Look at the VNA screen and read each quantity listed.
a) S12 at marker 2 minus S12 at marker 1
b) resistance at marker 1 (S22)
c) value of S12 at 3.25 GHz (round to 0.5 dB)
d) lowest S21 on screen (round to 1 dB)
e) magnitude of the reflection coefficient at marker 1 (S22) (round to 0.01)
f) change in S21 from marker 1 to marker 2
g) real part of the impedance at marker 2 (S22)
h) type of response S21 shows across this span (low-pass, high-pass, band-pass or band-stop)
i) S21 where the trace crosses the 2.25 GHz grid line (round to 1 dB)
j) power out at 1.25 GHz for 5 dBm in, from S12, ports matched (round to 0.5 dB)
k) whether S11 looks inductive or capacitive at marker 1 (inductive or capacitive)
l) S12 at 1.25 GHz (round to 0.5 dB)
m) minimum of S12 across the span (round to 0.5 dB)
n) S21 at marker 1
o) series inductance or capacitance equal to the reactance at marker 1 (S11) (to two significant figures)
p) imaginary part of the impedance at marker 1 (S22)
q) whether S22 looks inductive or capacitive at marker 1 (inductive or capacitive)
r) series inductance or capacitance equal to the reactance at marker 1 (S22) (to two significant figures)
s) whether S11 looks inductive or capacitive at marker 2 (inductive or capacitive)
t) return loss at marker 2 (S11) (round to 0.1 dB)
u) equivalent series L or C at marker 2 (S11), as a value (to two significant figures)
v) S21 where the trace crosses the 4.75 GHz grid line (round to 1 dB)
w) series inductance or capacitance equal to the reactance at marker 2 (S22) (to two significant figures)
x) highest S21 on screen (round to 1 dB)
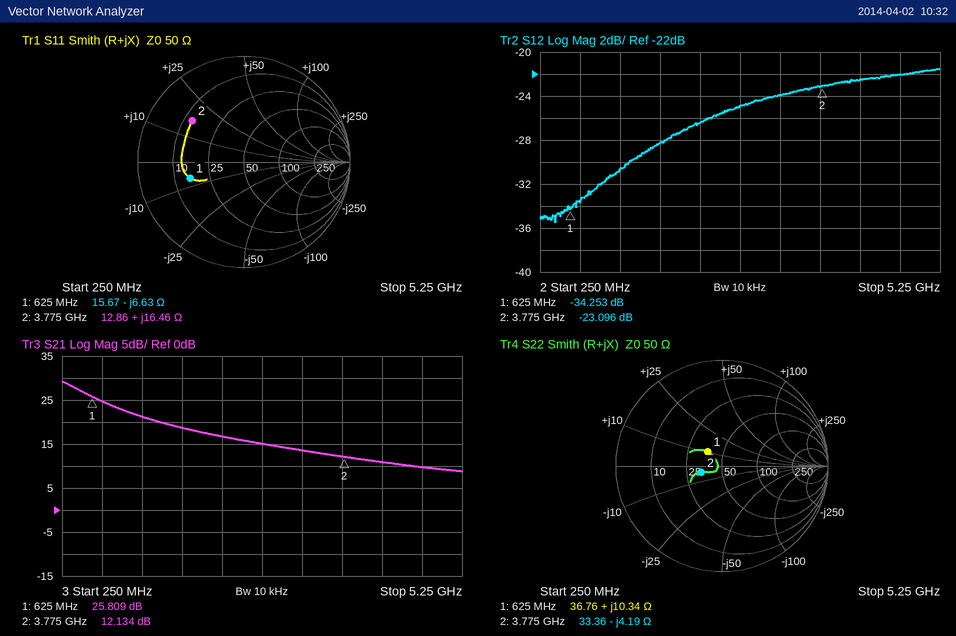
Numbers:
11.157 dB
36.76 Ω
-24.0 dB
9 dB
0.19
-13.675 dB
33.36 Ω
low-pass
17 dB
-25.5 dBm
capacitive
-30.5 dB
-35.5 dB
25.809 dB
38 pF
+10.34 Ω
inductive
2.6 nH
inductive
4.1 dB
690 pH
10 dB
10 pF
29 dB
